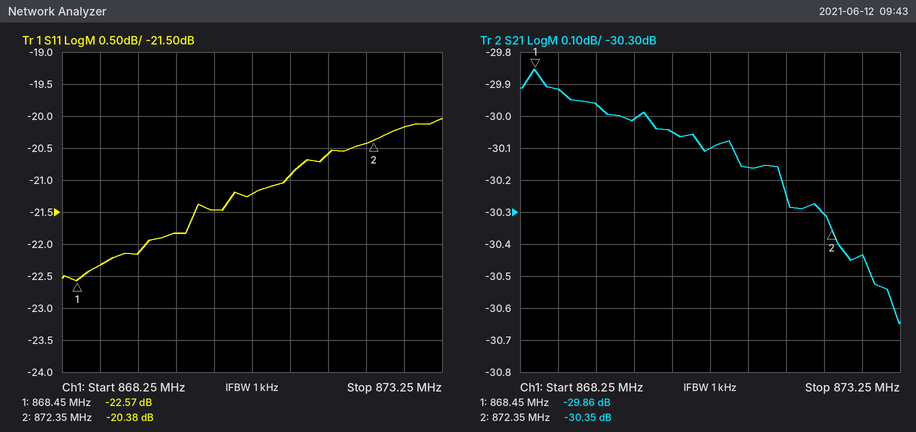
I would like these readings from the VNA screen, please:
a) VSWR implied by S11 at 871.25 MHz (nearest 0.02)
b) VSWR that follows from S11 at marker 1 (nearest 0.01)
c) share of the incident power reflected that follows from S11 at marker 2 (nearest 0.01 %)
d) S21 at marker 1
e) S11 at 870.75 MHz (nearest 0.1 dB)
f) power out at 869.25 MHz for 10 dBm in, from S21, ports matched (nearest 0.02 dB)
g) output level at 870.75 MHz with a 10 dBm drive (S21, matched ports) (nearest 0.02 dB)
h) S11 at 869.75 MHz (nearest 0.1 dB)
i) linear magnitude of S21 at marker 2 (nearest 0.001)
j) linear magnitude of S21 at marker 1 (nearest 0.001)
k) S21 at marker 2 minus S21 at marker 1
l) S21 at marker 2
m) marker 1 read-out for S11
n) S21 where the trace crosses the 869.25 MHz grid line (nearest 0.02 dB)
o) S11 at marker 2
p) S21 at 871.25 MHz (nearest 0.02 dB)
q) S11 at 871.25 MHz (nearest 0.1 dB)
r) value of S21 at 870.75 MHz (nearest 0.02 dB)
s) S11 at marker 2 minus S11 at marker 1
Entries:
1.20
1.16
0.92 %
-29.86 dB
-21.2 dB
-19.96 dBm
-20.10 dBm
-21.8 dB
0.030
0.032
-0.49 dB
-30.35 dB
-22.57 dB
-29.96 dB
-20.38 dB
-30.16 dB
-20.9 dB
-30.10 dB
2.19 dB
